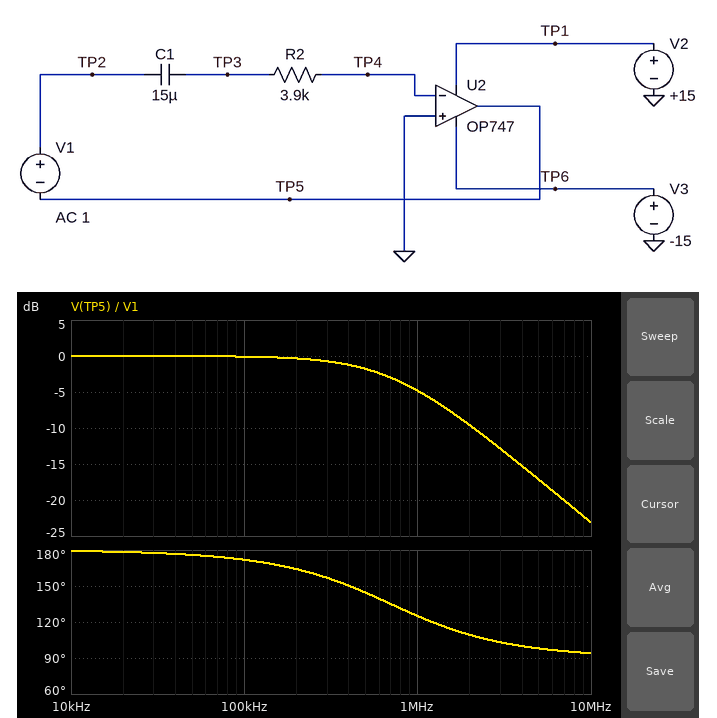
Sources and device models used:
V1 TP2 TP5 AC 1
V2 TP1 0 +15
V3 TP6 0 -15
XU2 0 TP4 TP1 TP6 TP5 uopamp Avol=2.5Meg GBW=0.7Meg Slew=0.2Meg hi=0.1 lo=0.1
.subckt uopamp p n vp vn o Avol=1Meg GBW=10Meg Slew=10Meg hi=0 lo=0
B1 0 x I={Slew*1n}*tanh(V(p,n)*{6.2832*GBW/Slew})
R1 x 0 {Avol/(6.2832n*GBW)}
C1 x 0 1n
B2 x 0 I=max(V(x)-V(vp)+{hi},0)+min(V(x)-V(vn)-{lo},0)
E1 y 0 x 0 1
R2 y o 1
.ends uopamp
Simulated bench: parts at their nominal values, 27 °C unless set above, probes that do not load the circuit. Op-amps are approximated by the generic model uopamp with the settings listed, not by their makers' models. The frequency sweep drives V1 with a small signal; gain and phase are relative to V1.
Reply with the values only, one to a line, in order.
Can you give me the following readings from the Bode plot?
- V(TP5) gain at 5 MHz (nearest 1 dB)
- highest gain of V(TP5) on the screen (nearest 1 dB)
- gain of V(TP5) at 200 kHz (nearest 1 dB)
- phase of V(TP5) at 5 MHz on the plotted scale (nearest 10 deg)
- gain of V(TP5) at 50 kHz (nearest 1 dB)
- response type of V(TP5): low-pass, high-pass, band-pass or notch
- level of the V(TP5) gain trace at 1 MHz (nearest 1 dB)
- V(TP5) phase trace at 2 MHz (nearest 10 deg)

-17 dB
0 dB
0 dB
100 deg
0 dB
low-pass
-5 dB
110 deg
